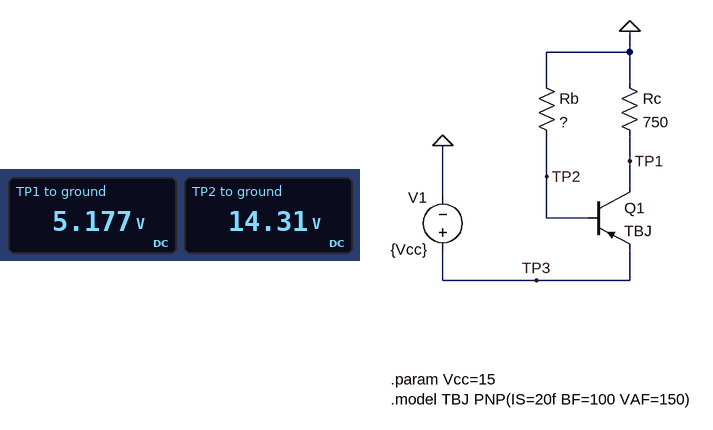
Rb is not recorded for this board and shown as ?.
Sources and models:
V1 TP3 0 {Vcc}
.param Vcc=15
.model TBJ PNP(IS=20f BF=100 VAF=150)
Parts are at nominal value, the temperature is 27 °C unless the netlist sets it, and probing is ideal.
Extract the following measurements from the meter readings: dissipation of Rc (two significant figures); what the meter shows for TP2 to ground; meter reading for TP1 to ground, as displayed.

36 mW
14.31 V
5.177 V
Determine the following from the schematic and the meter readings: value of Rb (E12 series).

220 kΩ
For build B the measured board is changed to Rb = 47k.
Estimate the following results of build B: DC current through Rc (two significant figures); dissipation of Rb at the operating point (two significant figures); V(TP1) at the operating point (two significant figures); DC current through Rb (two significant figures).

20 mA
4.3 mW
15 V
300 µA
